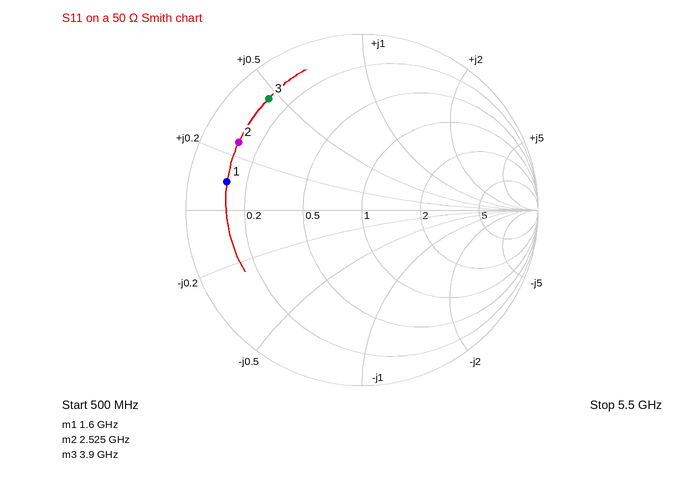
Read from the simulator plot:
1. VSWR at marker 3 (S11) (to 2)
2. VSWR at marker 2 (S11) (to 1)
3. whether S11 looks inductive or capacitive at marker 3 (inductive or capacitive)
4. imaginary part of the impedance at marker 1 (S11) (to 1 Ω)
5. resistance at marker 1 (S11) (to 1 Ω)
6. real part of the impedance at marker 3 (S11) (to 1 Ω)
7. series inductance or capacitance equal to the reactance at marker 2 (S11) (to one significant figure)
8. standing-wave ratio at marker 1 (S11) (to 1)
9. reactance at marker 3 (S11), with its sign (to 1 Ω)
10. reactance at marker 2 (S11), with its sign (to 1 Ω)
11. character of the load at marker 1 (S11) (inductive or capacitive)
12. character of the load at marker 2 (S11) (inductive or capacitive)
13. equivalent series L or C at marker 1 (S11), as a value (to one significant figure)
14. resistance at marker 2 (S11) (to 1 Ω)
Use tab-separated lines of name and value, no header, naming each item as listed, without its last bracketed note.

VSWR at marker 3 (S11)	10
VSWR at marker 2 (S11)	9
whether S11 looks inductive or capacitive at marker 3	inductive
imaginary part of the impedance at marker 1 (S11)	+5 Ω
resistance at marker 1 (S11)	6 Ω
real part of the impedance at marker 3 (S11)	6 Ω
series inductance or capacitance equal to the reactance at marker 2 (S11)	800 pH
standing-wave ratio at marker 1 (S11)	8
reactance at marker 3 (S11), with its sign	+23 Ω
reactance at marker 2 (S11), with its sign	+13 Ω
character of the load at marker 1 (S11)	inductive
character of the load at marker 2 (S11)	inductive
equivalent series L or C at marker 1 (S11), as a value	500 pH
resistance at marker 2 (S11)	6 Ω
